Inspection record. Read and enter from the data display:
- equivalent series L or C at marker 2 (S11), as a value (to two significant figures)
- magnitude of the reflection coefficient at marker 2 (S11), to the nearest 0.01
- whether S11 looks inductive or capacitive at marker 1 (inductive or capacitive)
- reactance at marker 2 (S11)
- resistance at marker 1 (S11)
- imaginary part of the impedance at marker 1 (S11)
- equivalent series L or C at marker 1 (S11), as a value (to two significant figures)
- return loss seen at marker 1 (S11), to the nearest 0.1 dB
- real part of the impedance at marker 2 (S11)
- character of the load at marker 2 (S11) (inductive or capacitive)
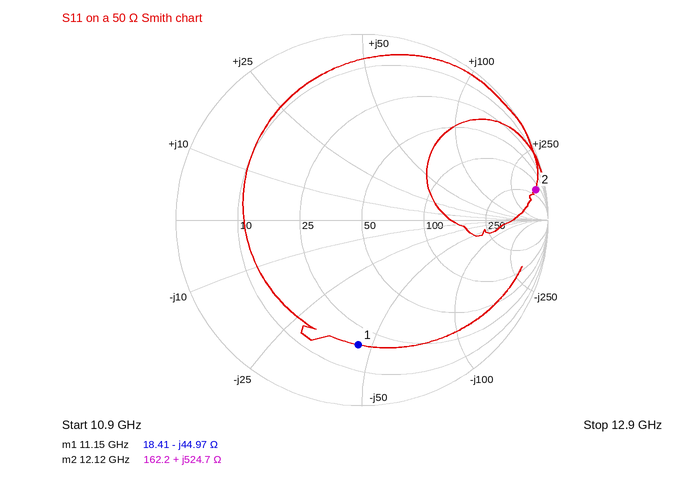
6.9 nH
0.95
capacitive
+524.7 Ω
18.41 Ω
-44.97 Ω
320 fF
3.5 dB
162.2 Ω
inductive
